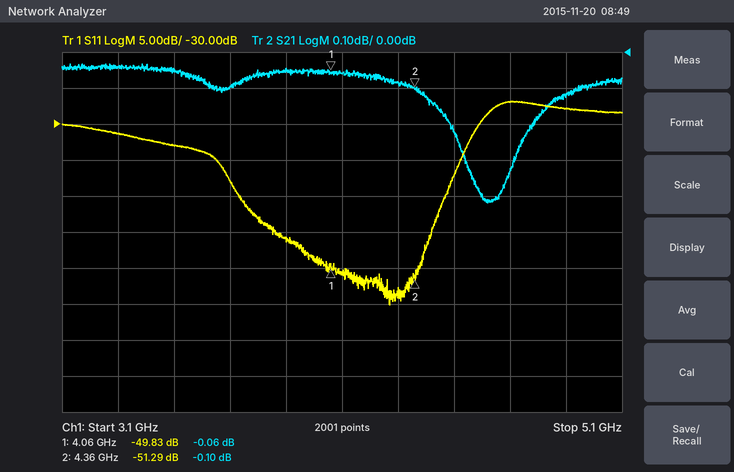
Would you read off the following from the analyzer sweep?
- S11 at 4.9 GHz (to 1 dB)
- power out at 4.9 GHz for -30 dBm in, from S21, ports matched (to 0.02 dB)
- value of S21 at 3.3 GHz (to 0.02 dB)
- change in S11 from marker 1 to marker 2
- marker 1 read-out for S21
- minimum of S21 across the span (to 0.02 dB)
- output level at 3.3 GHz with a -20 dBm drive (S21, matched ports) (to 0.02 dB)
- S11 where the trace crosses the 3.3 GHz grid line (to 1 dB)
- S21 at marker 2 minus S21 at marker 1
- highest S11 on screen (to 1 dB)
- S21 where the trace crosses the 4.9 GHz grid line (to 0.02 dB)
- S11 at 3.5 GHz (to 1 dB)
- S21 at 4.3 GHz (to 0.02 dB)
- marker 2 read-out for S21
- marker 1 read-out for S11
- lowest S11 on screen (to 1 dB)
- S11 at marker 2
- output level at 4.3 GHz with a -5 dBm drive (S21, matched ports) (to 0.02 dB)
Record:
-28 dB
-30.12 dBm
-0.04 dB
-1.46 dB
-0.06 dB
-0.42 dB
-20.04 dBm
-31 dB
-0.04 dB
-27 dB
-0.12 dB
-33 dB
-0.08 dB
-0.10 dB
-49.83 dB
-55 dB
-51.29 dB
-5.08 dBm
